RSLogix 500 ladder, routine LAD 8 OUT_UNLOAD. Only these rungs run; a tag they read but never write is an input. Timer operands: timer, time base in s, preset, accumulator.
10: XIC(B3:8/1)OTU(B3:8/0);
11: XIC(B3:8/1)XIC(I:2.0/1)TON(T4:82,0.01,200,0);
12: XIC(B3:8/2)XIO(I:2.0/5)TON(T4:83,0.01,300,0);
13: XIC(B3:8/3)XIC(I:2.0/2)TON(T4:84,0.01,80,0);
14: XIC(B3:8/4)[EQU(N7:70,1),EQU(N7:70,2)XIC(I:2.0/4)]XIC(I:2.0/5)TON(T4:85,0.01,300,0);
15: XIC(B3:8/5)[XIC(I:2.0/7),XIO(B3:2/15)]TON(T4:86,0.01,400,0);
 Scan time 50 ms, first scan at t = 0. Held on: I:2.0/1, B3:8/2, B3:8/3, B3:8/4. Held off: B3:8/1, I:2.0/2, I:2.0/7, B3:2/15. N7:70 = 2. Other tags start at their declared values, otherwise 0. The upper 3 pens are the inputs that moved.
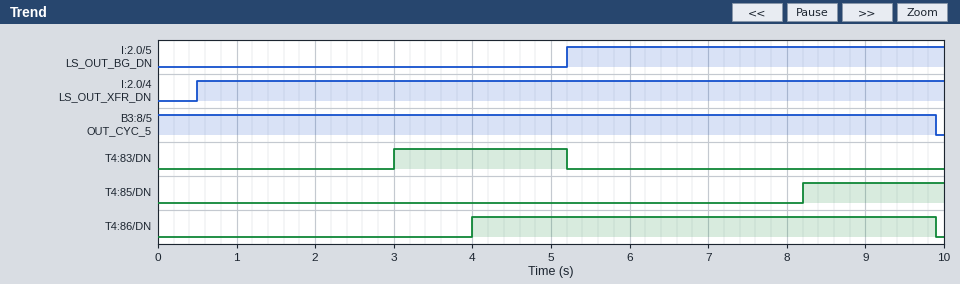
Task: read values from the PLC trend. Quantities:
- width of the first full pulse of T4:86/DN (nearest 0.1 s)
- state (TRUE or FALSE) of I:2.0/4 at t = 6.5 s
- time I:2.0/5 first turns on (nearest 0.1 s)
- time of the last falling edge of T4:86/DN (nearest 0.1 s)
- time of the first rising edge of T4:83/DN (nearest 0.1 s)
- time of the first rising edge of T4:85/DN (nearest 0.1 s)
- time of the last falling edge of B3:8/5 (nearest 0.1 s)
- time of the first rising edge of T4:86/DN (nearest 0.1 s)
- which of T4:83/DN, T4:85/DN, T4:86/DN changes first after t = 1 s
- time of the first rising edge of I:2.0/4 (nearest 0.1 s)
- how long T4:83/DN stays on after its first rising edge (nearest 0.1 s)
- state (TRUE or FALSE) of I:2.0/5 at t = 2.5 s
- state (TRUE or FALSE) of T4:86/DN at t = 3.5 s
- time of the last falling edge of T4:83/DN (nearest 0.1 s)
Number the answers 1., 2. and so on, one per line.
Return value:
1. 5.9 s
2. TRUE
3. 5.2 s
4. 9.9 s
5. 3.0 s
6. 8.2 s
7. 9.9 s
8. 4.0 s
9. T4:83/DN
10. 0.5 s
11. 2.2 s
12. FALSE
13. FALSE
14. 5.2 s
